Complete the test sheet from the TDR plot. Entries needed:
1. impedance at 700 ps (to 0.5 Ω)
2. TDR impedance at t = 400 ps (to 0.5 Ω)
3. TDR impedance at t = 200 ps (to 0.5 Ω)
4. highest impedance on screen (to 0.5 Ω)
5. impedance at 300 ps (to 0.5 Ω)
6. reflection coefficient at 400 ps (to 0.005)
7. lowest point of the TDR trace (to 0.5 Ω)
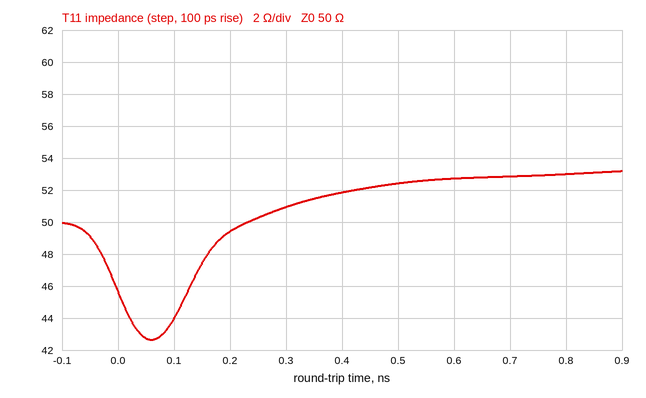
53.0 Ω
52.0 Ω
49.5 Ω
53.0 Ω
51.0 Ω
+0.020
42.5 Ω
